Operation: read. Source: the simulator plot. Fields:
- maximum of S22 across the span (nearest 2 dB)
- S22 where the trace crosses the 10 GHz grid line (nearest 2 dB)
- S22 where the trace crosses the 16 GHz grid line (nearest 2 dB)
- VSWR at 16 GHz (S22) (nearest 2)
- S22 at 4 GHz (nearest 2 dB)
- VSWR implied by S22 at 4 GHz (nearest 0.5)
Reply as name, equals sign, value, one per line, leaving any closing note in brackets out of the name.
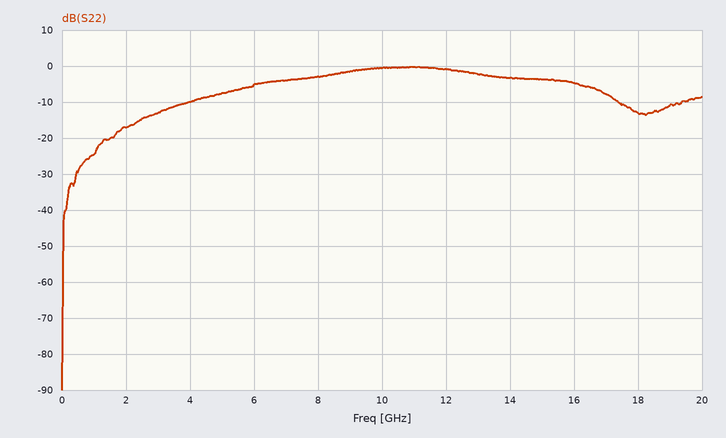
maximum of S22 across the span = 0 dB
S22 where the trace crosses the 10 GHz grid line = 0 dB
S22 where the trace crosses the 16 GHz grid line = -4 dB
VSWR at 16 GHz (S22) = 4
S22 at 4 GHz = -10 dB
VSWR implied by S22 at 4 GHz = 2.0
